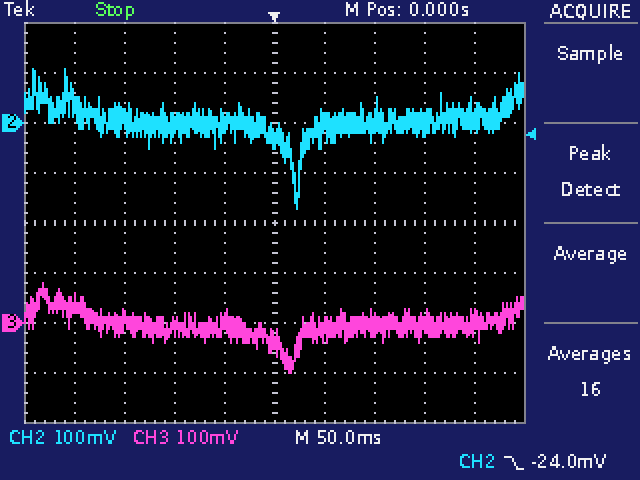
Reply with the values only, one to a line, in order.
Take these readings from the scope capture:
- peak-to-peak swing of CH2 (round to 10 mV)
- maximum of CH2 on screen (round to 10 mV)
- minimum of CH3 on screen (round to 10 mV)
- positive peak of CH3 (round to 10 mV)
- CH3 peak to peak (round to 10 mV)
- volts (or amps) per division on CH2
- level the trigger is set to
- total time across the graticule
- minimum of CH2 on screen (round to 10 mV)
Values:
280 mV
110 mV
-100 mV
80 mV
180 mV
100 mV
-24.0 mV
500 ms
-170 mV
